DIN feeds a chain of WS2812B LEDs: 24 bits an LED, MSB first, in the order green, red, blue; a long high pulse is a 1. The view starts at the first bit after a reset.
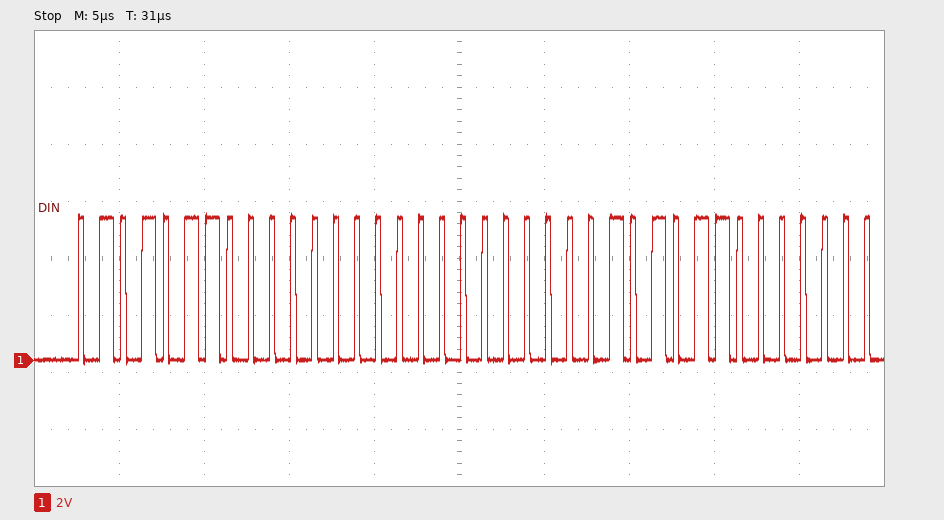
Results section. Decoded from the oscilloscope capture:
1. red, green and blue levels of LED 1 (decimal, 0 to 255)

0, 86, 0
